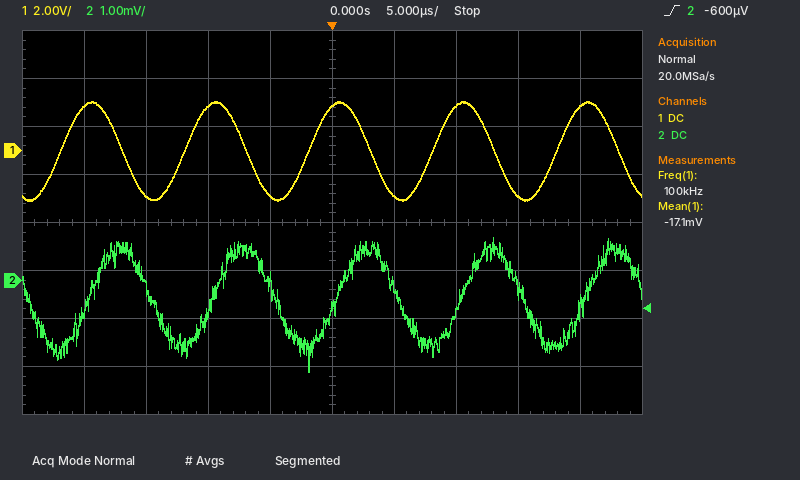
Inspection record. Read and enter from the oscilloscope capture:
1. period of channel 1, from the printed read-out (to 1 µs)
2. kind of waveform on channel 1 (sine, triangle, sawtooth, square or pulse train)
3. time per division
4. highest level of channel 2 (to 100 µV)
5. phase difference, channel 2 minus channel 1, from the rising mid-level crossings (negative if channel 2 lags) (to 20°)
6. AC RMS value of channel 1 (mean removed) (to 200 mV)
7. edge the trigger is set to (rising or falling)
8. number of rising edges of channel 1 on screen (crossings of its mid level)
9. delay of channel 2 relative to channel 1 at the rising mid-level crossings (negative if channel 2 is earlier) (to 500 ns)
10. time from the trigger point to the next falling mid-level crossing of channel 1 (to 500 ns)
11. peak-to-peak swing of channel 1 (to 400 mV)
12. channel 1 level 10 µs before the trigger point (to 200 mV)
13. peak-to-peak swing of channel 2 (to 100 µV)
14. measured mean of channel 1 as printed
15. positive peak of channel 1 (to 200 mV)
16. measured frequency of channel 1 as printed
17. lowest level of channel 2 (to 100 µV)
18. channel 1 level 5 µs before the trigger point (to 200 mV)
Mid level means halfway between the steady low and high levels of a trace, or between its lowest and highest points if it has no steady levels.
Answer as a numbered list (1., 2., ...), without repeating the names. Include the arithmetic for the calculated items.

1. 1 / 100 kHz ≈ 10 µs
2. sine
3. 5 µs
4. 900 µV
5. -80°
6. 4.0 V / (2√2) ≈ 1.4 V
7. rising
8. 5
9. +2.0 µs
10. 3.0 µs
11. 4.0 V
12. 1.8 V
13. 900 µV − (-1.9 mV) = 2.8 mV
14. -17.1 mV
15. 2.0 V
16. 100 kHz
17. -1.9 mV
18. -1.8 V
